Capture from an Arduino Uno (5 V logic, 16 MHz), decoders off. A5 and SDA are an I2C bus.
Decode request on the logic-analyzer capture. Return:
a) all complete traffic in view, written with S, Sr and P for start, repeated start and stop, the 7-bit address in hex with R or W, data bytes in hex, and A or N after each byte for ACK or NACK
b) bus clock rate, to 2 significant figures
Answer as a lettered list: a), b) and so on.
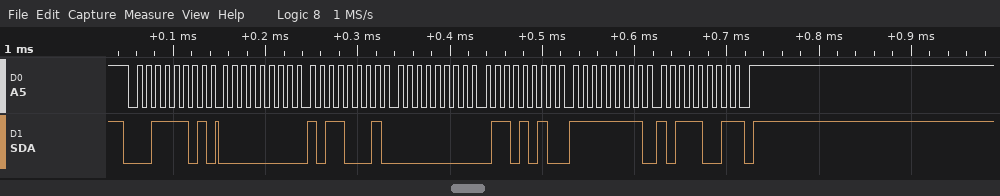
a) S 1ER A 00 A B1 A 00 A 6A A FF A B9 N P
b) 100 kHz
